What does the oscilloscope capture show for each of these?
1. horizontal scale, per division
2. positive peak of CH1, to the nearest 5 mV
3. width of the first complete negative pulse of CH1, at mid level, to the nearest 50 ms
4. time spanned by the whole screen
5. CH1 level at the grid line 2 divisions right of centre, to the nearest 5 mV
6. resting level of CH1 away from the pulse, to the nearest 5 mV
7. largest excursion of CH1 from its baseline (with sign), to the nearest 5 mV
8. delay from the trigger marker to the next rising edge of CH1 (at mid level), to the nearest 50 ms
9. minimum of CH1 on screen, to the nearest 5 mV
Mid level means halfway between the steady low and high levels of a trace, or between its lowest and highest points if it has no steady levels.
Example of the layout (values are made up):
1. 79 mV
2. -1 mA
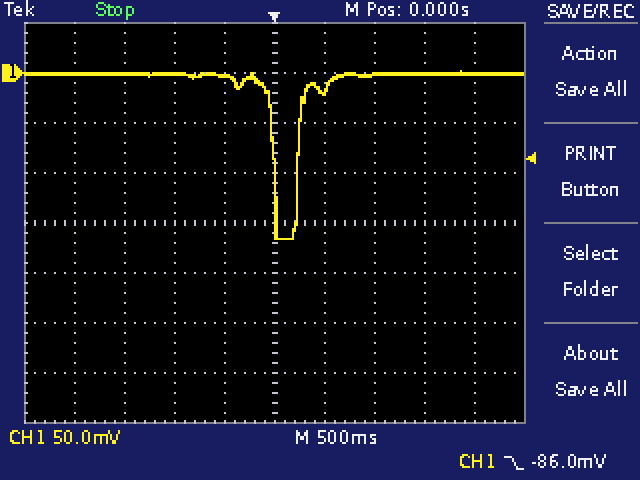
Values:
1. 500 ms
2. 0 mV
3. 250 ms
4. 5 s
5. 0 mV
6. 0 mV
7. -165 mV
8. 250 ms
9. -165 mV
